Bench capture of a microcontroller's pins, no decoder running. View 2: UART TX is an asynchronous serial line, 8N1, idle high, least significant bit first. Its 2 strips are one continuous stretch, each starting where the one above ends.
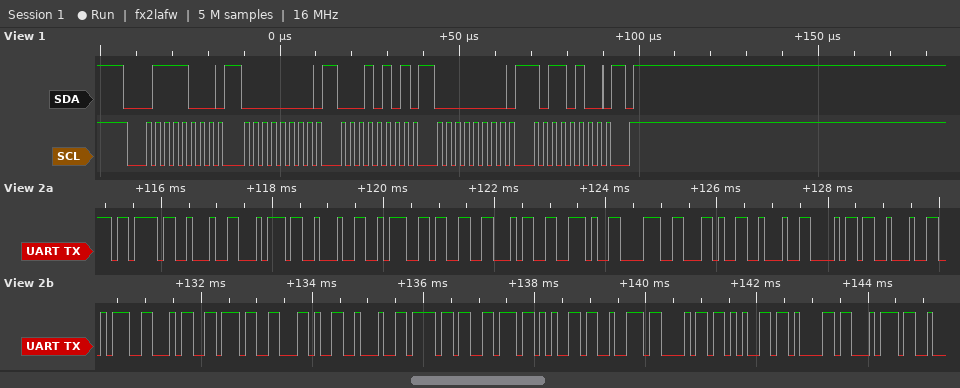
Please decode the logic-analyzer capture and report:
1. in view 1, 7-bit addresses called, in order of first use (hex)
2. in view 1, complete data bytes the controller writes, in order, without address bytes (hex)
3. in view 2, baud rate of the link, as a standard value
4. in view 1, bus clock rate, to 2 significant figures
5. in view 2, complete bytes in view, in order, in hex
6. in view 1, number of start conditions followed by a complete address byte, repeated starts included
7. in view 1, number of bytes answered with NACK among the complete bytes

0x3C
00 15 00 B4
9600 baud
400 kHz
0x7B 0x22 0x74 0x22 0x3A 0x33 0x34 0x2E 0x38 0x2C 0x22 0x68 0x22 0x3A 0x34 0x37 0x2C 0x22 0x6F 0x76 0x65 0x72 0x68 0x65 0x61 0x74
1
0
